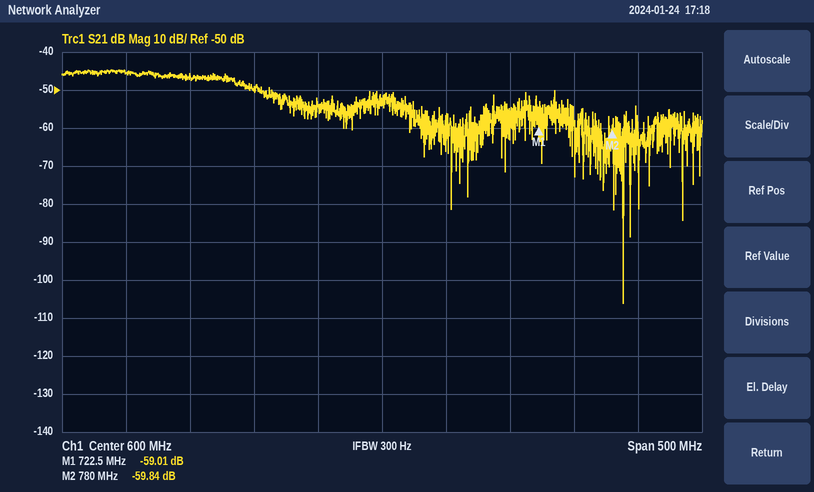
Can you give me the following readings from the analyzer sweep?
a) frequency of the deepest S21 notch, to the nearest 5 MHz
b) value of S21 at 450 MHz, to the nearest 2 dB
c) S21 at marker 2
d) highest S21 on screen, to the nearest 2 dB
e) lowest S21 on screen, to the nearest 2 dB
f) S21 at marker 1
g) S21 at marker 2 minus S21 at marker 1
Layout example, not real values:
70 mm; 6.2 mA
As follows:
790 MHz; -46 dB; -59.84 dB; -44 dB; -106 dB; -59.01 dB; -0.83 dB
